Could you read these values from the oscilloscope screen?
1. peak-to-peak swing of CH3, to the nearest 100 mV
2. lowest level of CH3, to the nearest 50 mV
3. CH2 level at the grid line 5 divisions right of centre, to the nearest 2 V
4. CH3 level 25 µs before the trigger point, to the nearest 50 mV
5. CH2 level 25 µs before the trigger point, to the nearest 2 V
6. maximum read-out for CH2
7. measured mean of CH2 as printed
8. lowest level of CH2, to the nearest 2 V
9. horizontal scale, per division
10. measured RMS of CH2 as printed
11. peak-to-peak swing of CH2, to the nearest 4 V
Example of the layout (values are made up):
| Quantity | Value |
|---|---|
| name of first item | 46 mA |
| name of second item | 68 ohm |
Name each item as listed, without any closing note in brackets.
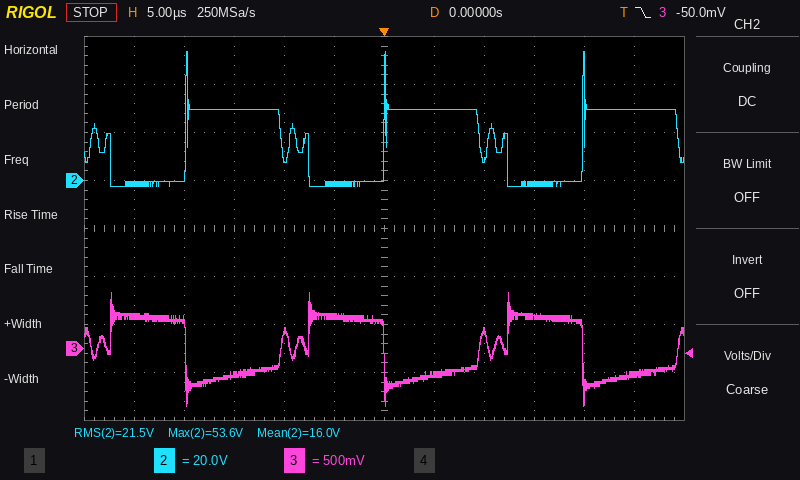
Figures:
| Quantity | Value |
|---|---|
| peak-to-peak swing of CH3, to the nearest 100 mV | 1.20 V |
| lowest level of CH3, to the nearest 50 mV | -600 mV |
| CH2 level at the grid line 5 divisions right of centre, to the nearest 2 V | 30 V |
| CH3 level 25 µs before the trigger point, to the nearest 50 mV | 350 mV |
| CH2 level 25 µs before the trigger point, to the nearest 2 V | -2 V |
| maximum read-out for CH2 | 53.6 V |
| measured mean of CH2 as printed | 16.0 V |
| lowest level of CH2, to the nearest 2 V | -2 V |
| horizontal scale, per division | 5 µs |
| measured RMS of CH2 as printed | 21.5 V |
| peak-to-peak swing of CH2, to the nearest 4 V | 56 V |
